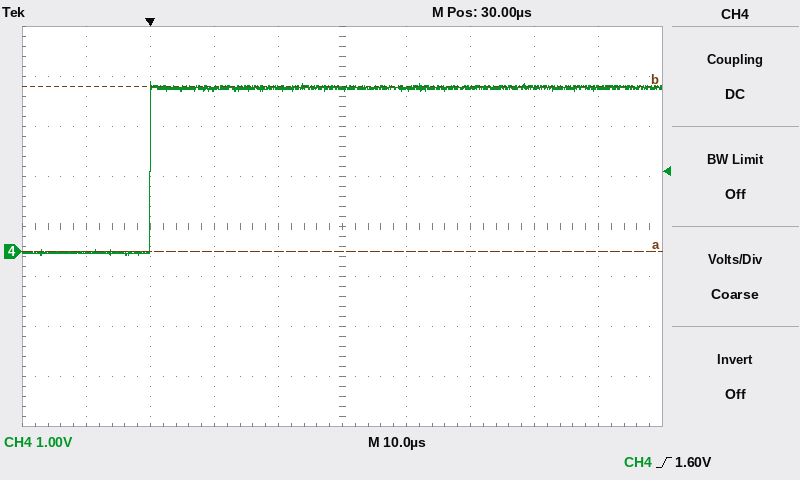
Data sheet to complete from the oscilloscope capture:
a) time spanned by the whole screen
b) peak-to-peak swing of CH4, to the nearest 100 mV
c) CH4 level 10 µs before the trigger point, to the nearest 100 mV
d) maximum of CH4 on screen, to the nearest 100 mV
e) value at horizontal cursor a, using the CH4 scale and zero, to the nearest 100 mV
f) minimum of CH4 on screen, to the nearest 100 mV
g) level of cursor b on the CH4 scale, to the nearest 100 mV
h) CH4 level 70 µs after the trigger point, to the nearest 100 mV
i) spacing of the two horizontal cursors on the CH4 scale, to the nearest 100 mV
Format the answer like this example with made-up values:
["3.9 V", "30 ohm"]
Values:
["100 µs", "3.5 V", "0.0 V", "3.4 V", "0.0 V", "-100 mV", "3.3 V", "3.3 V", "3.3 V"]
